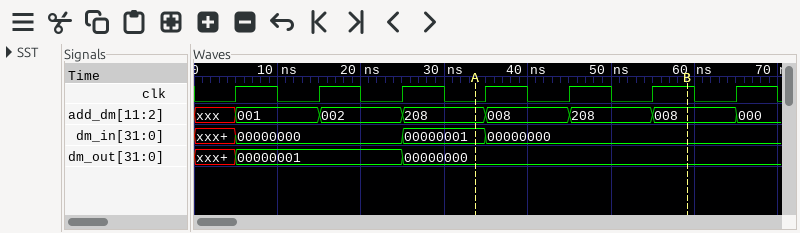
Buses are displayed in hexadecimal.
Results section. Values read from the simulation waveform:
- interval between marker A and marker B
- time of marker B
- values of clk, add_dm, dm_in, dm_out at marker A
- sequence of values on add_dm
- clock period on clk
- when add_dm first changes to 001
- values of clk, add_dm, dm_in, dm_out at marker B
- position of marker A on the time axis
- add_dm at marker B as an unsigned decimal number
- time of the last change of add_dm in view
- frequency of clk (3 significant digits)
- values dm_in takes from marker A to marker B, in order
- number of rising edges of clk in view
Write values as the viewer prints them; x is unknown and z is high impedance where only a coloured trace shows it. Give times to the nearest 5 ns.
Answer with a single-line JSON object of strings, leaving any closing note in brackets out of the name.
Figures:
{"interval between marker A and marker B": "25 ns", "time of marker B": "60 ns", "values of clk, add_dm, dm_in, dm_out at marker A": "clk=0, add_dm=208, dm_in=00000001, dm_out=00000000", "sequence of values on add_dm": "xxx, 001, 002, 208, 008, 208, 008, 000", "clock period on clk": "10 ns", "when add_dm first changes to 001": "5 ns", "values of clk, add_dm, dm_in, dm_out at marker B": "clk=1, add_dm=008, dm_in=00000000, dm_out=00000000", "position of marker A on the time axis": "35 ns", "add_dm at marker B as an unsigned decimal number": "8", "time of the last change of add_dm in view": "65 ns", "frequency of clk": "100 MHz", "values dm_in takes from marker A to marker B, in order": "00000001, 00000000", "number of rising edges of clk in view": "7"}
